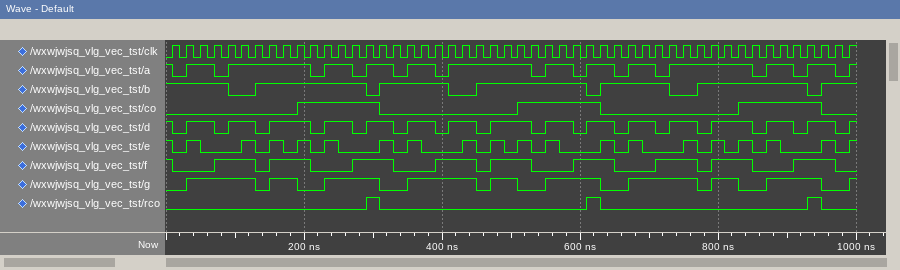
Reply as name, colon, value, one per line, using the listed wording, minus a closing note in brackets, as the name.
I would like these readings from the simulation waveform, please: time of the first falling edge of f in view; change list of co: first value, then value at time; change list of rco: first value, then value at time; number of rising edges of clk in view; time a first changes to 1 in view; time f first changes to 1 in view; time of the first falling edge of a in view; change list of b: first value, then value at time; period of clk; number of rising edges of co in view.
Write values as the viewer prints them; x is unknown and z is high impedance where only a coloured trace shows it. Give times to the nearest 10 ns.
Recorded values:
time of the first falling edge of f in view: 10 ns
change list of co: first value, then value at time: 0, 1 at 190 ns, 0 at 310 ns, 1 at 510 ns, 0 at 630 ns, 1 at 830 ns, 0 at 950 ns
change list of rco: first value, then value at time: 0, 1 at 290 ns, 0 at 310 ns, 1 at 610 ns, 0 at 630 ns, 1 at 930 ns, 0 at 950 ns
number of rising edges of clk in view: 50
time a first changes to 1 in view: 30 ns
time f first changes to 1 in view: 70 ns
time of the first falling edge of a in view: 10 ns
change list of b: first value, then value at time: 1, 0 at 90 ns, 1 at 130 ns, 0 at 290 ns, 1 at 310 ns, 0 at 410 ns, 1 at 450 ns, 0 at 610 ns, 1 at 630 ns, 0 at 730 ns, 1 at 770 ns, 0 at 930 ns, 1 at 950 ns
period of clk: 20 ns
number of rising edges of co in view: 3
